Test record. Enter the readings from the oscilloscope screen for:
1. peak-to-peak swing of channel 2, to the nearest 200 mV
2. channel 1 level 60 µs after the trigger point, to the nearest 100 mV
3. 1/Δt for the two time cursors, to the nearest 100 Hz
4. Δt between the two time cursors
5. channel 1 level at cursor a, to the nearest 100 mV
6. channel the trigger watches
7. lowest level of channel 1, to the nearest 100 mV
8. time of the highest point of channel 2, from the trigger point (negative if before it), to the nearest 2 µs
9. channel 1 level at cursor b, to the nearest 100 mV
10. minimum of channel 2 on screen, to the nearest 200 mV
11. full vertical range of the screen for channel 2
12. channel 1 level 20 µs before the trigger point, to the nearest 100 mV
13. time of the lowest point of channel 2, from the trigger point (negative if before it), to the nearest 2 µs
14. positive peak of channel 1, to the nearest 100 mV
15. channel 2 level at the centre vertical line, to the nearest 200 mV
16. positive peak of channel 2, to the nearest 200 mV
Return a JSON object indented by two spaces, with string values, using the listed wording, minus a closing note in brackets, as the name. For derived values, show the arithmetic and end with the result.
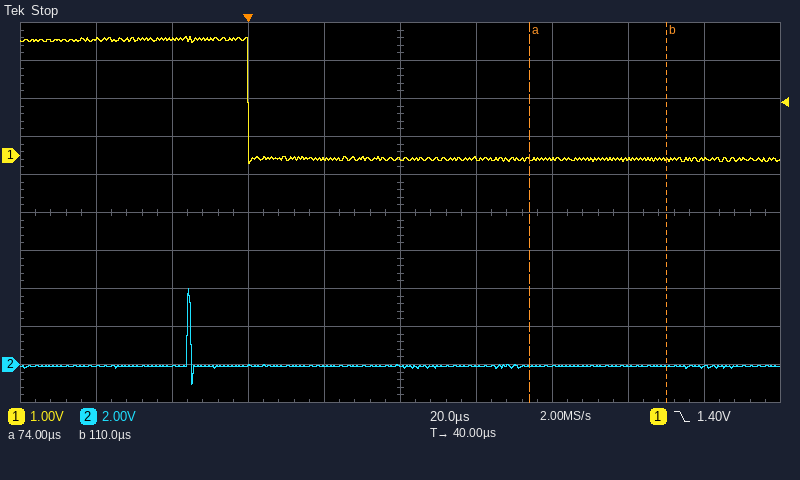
{
  "peak-to-peak swing of channel 2, to the nearest 200 mV": "4.0 V − (-1.0 V) = 5.0 V",
  "channel 1 level 60 µs after the trigger point, to the nearest 100 mV": "-100 mV",
  "1/Δt for the two time cursors, to the nearest 100 Hz": "1 / 36 µs ≈ 27.8 kHz",
  "Δt between the two time cursors": "110 µs − (74 µs) = 36 µs",
  "channel 1 level at cursor a, to the nearest 100 mV": "-100 mV",
  "channel the trigger watches": "channel 1",
  "lowest level of channel 1, to the nearest 100 mV": "-200 mV",
  "time of the highest point of channel 2, from the trigger point (negative if before it), to the nearest 2 µs": "-16 µs",
  "channel 1 level at cursor b, to the nearest 100 mV": "-100 mV",
  "minimum of channel 2 on screen, to the nearest 200 mV": "-1.0 V",
  "full vertical range of the screen for channel 2": "20 V",
  "channel 1 level 20 µs before the trigger point, to the nearest 100 mV": "3.1 V",
  "time of the lowest point of channel 2, from the trigger point (negative if before it), to the nearest 2 µs": "-14 µs",
  "positive peak of channel 1, to the nearest 100 mV": "3.1 V",
  "channel 2 level at the centre vertical line, to the nearest 200 mV": "0.0 V",
  "positive peak of channel 2, to the nearest 200 mV": "4.0 V"
}
